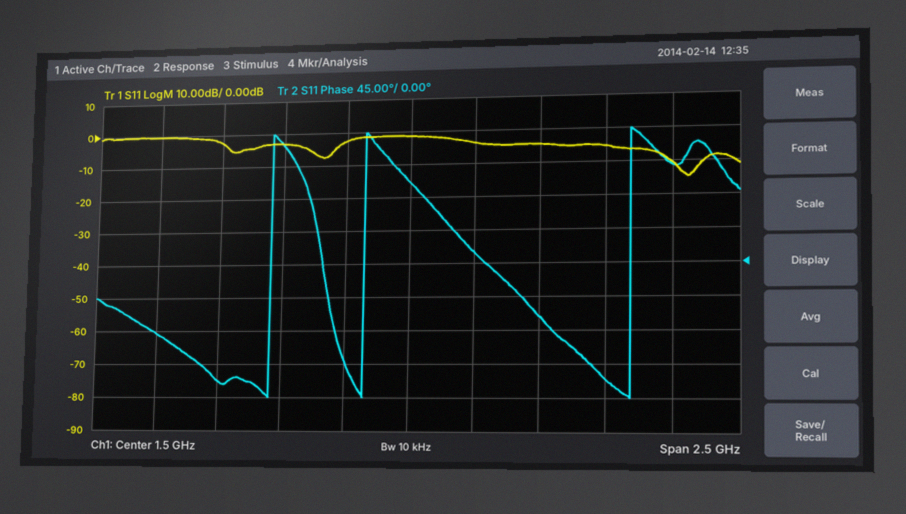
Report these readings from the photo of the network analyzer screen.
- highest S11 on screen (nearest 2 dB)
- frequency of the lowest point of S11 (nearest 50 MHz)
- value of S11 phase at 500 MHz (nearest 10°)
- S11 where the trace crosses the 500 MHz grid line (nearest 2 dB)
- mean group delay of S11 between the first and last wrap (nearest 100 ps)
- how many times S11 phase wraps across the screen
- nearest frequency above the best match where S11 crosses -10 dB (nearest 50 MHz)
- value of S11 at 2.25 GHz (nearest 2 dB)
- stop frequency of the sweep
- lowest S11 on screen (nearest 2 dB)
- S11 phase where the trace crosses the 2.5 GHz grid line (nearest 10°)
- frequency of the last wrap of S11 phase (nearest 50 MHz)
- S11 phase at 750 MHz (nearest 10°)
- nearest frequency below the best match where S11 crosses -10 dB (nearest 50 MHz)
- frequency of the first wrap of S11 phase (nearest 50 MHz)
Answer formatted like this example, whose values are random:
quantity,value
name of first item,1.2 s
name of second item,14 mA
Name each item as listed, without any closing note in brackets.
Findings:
quantity,value
highest S11 on screen,0 dB
frequency of the lowest point of S11,2.55 GHz
value of S11 phase at 500 MHz,-90°
S11 where the trace crosses the 500 MHz grid line,0 dB
mean group delay of S11 between the first and last wrap,1.4 ns
how many times S11 phase wraps across the screen,3
nearest frequency above the best match where S11 crosses -10 dB,2.60 GHz
value of S11 at 2.25 GHz,-6 dB
stop frequency of the sweep,2.75 GHz
lowest S11 on screen,-14 dB
S11 phase where the trace crosses the 2.5 GHz grid line,130°
frequency of the last wrap of S11 phase,2.35 GHz
S11 phase at 750 MHz,-160°
nearest frequency below the best match where S11 crosses -10 dB,2.50 GHz
frequency of the first wrap of S11 phase,950 MHz
